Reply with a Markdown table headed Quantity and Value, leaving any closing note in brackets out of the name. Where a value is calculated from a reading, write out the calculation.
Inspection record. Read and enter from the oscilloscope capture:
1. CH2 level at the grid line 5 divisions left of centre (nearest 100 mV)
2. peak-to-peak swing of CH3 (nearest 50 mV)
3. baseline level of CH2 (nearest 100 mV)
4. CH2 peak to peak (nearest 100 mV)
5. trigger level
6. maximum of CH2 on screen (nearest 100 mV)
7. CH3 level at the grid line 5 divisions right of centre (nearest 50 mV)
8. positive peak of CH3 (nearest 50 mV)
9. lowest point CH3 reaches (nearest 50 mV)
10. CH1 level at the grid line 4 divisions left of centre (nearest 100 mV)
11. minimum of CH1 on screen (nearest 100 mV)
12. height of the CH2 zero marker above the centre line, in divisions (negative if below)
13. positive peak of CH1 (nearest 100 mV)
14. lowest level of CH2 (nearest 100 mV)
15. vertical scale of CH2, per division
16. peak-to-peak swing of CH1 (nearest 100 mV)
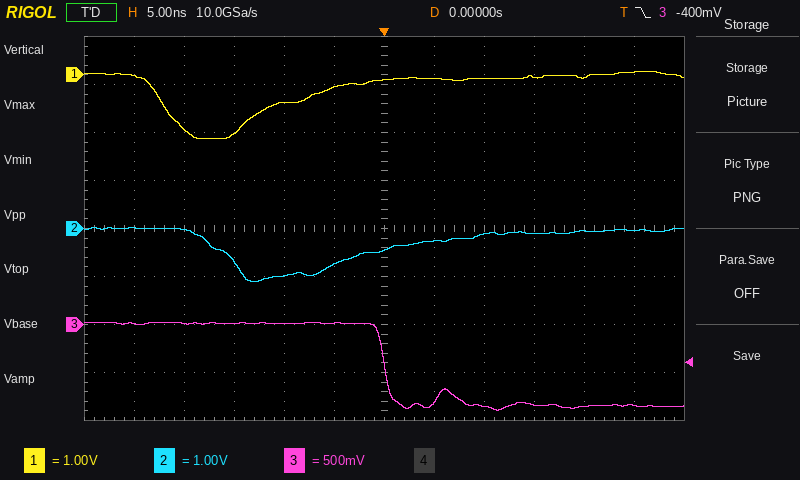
| Quantity | Value |
|---|---|
| CH2 level at the grid line 5 divisions left of centre | 0.0 V |
| peak-to-peak swing of CH3 | 0 mV − (-900 mV) = 900 mV |
| baseline level of CH2 | -100 mV |
| CH2 peak to peak | 0.0 V − (-1.1 V) = 1.1 V |
| trigger level | -400 mV |
| maximum of CH2 on screen | 0.0 V |
| CH3 level at the grid line 5 divisions right of centre | -850 mV |
| positive peak of CH3 | 0 mV |
| lowest point CH3 reaches | -900 mV |
| CH1 level at the grid line 4 divisions left of centre | -1.1 V |
| minimum of CH1 on screen | -1.3 V |
| height of the CH2 zero marker above the centre line, in divisions | 0.0 div |
| positive peak of CH1 | 100 mV |
| lowest level of CH2 | -1.1 V |
| vertical scale of CH2, per division | 1 V |
| peak-to-peak swing of CH1 | 100 mV − (-1.3 V) = 1.4 V |
